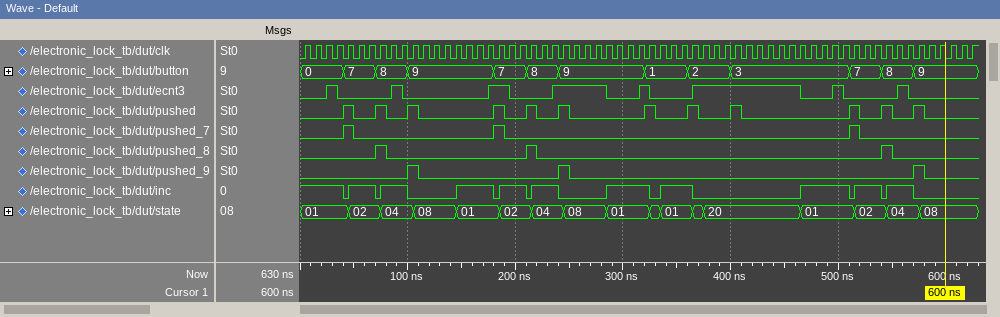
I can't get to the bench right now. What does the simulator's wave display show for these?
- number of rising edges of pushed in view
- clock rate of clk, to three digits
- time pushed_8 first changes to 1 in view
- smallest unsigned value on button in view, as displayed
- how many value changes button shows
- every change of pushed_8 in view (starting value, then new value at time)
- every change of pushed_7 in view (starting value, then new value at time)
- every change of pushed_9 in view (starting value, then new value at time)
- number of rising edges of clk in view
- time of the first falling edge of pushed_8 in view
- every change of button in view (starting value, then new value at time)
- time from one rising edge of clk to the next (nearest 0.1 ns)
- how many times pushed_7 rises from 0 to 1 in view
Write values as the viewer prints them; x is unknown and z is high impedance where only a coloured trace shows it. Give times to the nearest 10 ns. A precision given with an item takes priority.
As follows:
12
100 MHz
70 ns
0
12
0, 1 at 70 ns, 0 at 80 ns, 1 at 210 ns, 0 at 220 ns, 1 at 540 ns, 0 at 550 ns
0, 1 at 40 ns, 0 at 50 ns, 1 at 180 ns, 0 at 190 ns, 1 at 510 ns, 0 at 520 ns
0, 1 at 100 ns, 0 at 110 ns, 1 at 240 ns, 0 at 250 ns, 1 at 570 ns, 0 at 580 ns
63
80 ns
0, 7 at 40 ns, 8 at 70 ns, 9 at 100 ns, 7 at 180 ns, 8 at 210 ns, 9 at 240 ns, 1 at 320 ns, 2 at 360 ns, 3 at 400 ns, 7 at 510 ns, 8 at 540 ns, 9 at 570 ns
10 ns
3
